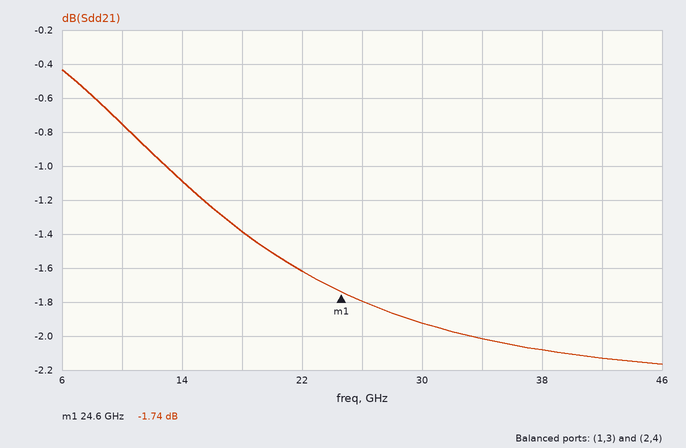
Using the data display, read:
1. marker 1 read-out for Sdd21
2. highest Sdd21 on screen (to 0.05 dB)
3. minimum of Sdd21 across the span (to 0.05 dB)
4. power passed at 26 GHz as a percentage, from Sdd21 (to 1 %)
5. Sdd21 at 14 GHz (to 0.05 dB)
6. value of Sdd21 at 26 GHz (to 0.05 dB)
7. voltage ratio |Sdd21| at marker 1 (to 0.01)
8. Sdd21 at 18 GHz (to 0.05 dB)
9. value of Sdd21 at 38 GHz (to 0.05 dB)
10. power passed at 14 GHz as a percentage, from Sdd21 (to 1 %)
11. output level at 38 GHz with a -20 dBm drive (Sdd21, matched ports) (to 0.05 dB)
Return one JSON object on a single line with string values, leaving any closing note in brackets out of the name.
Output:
{"marker 1 read-out for Sdd21": "-1.74 dB", "highest Sdd21 on screen": "-0.45 dB", "minimum of Sdd21 across the span": "-2.15 dB", "power passed at 26 GHz as a percentage, from Sdd21": "66 %", "Sdd21 at 14 GHz": "-1.10 dB", "value of Sdd21 at 26 GHz": "-1.80 dB", "voltage ratio |Sdd21| at marker 1": "0.82", "Sdd21 at 18 GHz": "-1.40 dB", "value of Sdd21 at 38 GHz": "-2.10 dB", "power passed at 14 GHz as a percentage, from Sdd21": "78 %", "output level at 38 GHz with a -20 dBm drive (Sdd21, matched ports)": "-22.10 dBm"}
